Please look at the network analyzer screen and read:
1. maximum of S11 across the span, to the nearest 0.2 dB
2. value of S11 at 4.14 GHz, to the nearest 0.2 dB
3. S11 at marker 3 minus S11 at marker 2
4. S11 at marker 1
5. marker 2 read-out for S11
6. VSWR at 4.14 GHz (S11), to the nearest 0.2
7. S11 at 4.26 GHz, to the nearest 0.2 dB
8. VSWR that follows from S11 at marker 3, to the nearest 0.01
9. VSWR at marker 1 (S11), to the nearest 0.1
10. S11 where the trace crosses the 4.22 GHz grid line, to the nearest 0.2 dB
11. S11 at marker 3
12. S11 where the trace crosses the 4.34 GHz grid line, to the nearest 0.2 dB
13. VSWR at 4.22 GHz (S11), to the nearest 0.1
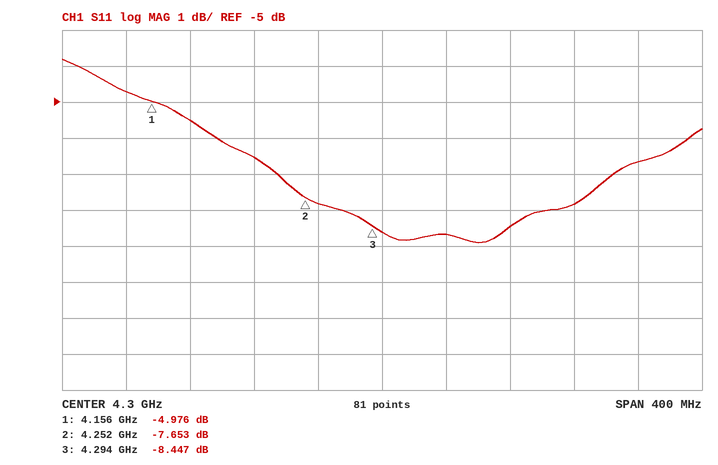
-3.8 dB
-4.8 dB
-0.794 dB
-4.976 dB
-7.653 dB
3.8
-7.8 dB
2.22
3.6
-6.6 dB
-8.447 dB
-8.6 dB
2.8
